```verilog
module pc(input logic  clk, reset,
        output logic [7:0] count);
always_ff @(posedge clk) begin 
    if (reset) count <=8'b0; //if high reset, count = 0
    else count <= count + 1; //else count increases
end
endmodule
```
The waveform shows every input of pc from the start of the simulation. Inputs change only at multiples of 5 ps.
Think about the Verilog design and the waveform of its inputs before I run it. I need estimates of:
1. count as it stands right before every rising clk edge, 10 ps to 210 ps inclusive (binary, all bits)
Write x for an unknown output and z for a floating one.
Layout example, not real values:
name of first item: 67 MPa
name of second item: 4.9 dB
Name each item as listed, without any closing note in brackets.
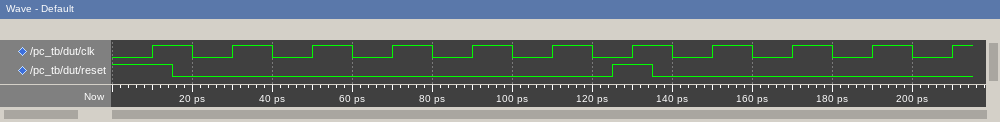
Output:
count as it stands right before every rising clk edge, 10 ps to 210 ps inclusive: x, 00000000, 00000001, 00000010, 00000011, 00000100, 00000101, 00000000, 00000001, 00000010, 00000011
